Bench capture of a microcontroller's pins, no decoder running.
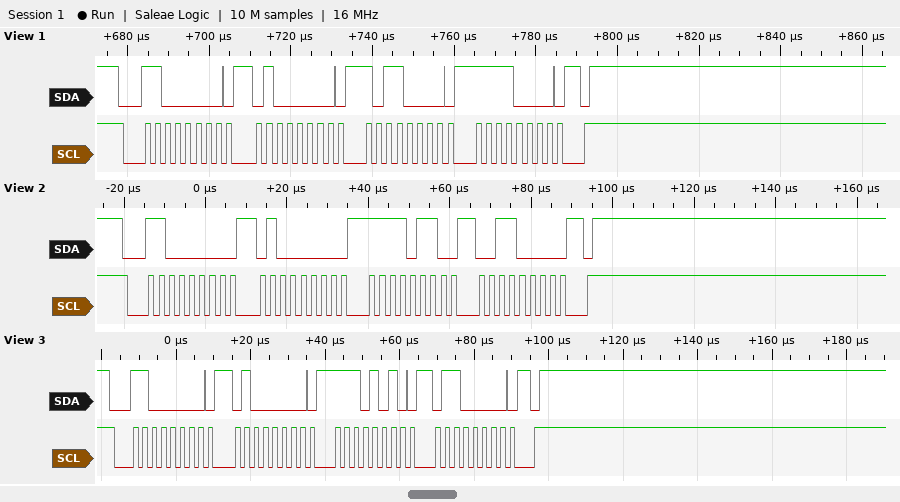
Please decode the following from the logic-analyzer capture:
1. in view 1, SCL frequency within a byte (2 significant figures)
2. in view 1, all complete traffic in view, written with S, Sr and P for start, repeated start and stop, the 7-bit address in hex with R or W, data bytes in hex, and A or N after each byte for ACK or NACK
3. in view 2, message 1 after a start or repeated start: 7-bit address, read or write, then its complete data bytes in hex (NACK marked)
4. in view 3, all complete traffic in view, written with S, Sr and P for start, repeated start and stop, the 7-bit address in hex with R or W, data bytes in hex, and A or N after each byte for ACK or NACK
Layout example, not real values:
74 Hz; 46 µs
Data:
400 kHz; S 60W A 40 A B0 A F0 A P; 0x60 write: 40 F6 30; S 60W A 40 A EA A 60 A P
